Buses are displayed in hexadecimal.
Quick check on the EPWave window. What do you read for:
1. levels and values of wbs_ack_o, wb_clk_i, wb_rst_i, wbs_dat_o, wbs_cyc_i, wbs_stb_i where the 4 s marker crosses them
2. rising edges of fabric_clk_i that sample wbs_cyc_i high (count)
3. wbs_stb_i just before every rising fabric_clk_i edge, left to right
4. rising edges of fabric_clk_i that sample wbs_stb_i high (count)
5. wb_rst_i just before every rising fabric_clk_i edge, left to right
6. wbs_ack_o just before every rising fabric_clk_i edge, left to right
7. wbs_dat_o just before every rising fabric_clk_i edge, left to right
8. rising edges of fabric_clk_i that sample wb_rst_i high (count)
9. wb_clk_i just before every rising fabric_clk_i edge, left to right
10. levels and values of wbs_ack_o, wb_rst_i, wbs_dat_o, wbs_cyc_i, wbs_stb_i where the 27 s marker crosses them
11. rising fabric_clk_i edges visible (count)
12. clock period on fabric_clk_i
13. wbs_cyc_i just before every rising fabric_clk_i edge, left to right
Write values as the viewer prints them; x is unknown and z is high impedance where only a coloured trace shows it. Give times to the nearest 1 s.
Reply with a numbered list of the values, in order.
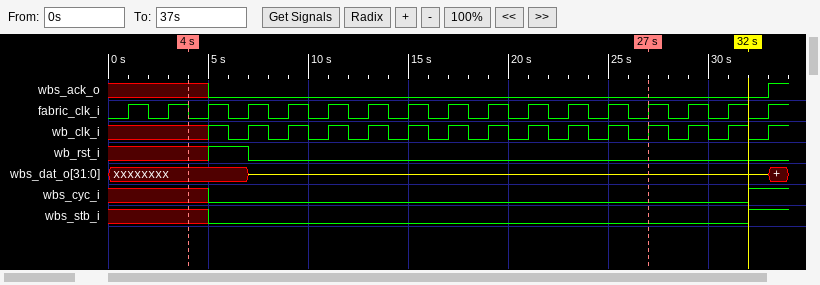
1. wbs_ack_o=x, wb_clk_i=x, wb_rst_i=x, wbs_dat_o=xxxxxxxx, wbs_cyc_i=x, wbs_stb_i=x
2. 1
3. x x x 0 0 0 0 0 0 0 0 0 0 0 0 0 1
4. 1
5. x x x 1 0 0 0 0 0 0 0 0 0 0 0 0 0
6. x x x 0 0 0 0 0 0 0 0 0 0 0 0 0 0
7. xxxxxxxx, xxxxxxxx, xxxxxxxx, xxxxxxxx, z, z, z, z, z, z, z, z, z, z, z, z, z
8. 1
9. x x x 0 0 0 0 0 0 0 0 0 0 0 0 0 0
10. wbs_ack_o=0, wb_rst_i=0, wbs_dat_o=z, wbs_cyc_i=0, wbs_stb_i=0
11. 17
12. 2 s
13. x x x 0 0 0 0 0 0 0 0 0 0 0 0 0 1
